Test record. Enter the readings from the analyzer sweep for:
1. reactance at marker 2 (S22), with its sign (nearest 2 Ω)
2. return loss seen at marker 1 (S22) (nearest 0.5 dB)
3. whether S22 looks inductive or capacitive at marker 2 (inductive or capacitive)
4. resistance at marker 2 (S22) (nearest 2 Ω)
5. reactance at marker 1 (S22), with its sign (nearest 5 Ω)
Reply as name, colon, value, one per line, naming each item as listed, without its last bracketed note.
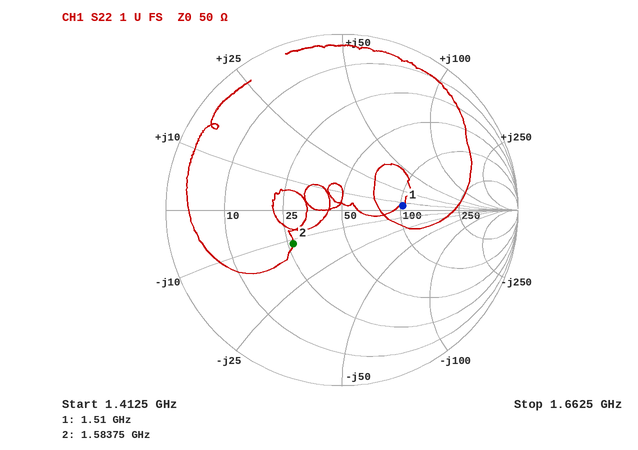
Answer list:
reactance at marker 2 (S22), with its sign: -12 Ω
return loss seen at marker 1 (S22): 9.0 dB
whether S22 looks inductive or capacitive at marker 2: capacitive
resistance at marker 2 (S22): 26 Ω
reactance at marker 1 (S22), with its sign: +5 Ω
